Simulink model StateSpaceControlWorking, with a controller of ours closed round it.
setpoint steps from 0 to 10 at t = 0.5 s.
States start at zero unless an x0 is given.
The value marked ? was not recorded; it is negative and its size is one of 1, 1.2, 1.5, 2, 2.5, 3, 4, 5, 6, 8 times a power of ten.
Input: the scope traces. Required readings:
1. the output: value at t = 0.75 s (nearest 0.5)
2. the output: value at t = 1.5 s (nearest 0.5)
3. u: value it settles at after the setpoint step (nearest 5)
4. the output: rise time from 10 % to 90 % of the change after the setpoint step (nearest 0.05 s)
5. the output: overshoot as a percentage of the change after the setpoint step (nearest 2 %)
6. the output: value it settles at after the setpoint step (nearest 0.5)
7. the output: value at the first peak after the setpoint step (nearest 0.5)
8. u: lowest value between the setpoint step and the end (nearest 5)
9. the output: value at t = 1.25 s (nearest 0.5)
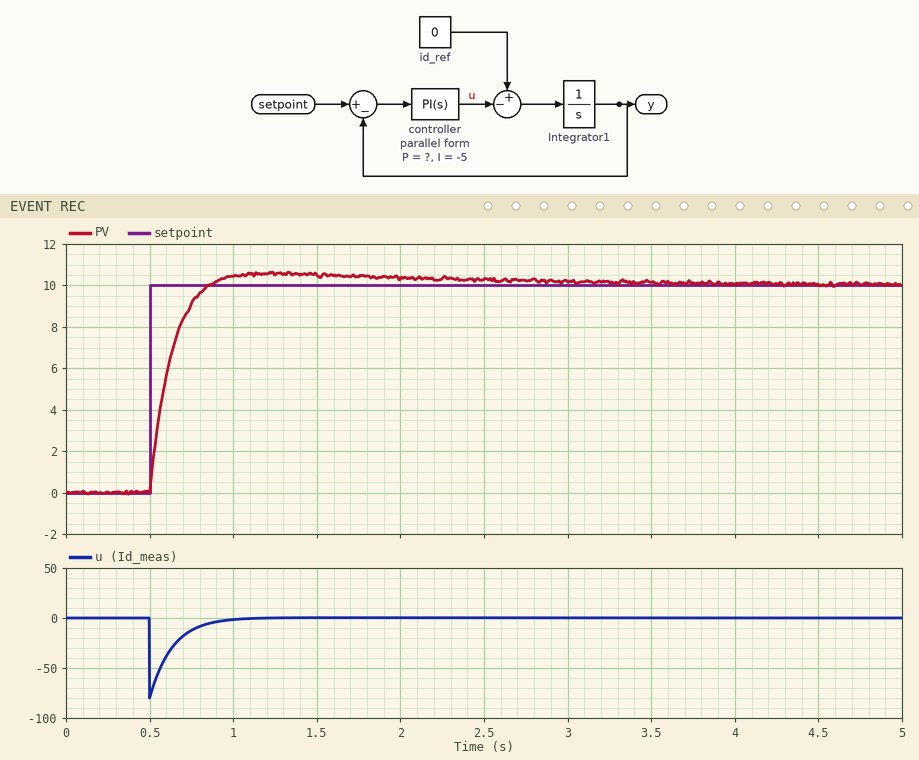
9.0
10.5
0
0.25 s
6 %
10.0
10.5
-80
10.5
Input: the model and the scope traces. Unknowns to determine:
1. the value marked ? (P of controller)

-8
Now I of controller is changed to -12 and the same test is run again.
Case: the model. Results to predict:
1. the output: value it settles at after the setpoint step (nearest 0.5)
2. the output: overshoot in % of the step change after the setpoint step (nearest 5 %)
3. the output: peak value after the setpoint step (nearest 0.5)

10.0
10 %
11.0
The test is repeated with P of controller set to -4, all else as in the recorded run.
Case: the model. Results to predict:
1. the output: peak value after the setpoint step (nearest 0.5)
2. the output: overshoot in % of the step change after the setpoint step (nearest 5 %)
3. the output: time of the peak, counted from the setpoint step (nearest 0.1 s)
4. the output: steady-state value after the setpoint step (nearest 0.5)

11.5
15 %
0.9 s
10.0
